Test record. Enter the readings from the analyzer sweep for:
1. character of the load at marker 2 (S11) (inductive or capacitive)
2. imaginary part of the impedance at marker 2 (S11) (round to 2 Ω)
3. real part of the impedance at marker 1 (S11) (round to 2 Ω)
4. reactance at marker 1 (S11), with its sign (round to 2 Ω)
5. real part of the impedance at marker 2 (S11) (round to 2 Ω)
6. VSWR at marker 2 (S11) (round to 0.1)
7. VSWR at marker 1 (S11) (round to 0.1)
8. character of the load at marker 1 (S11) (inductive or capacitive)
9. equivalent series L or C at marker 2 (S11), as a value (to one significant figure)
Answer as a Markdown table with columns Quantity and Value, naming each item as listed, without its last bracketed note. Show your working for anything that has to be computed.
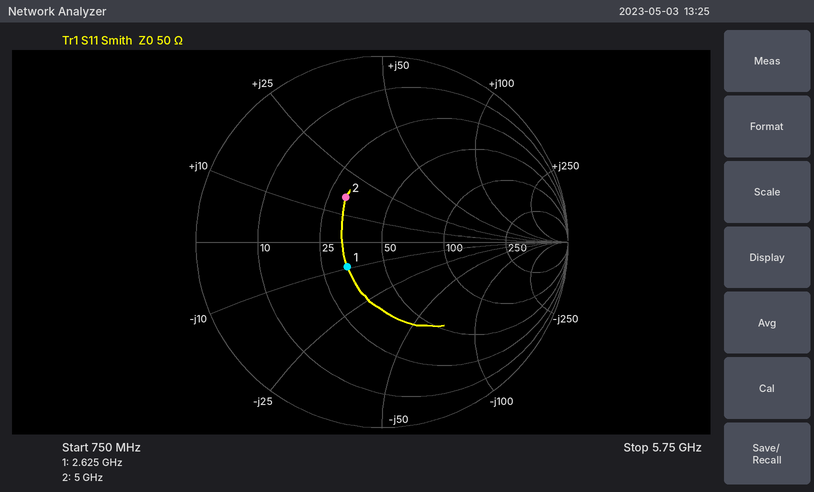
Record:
| Quantity | Value |
|---|---|
| character of the load at marker 2 (S11) | inductive |
| imaginary part of the impedance at marker 2 (S11) | +16 Ω |
| real part of the impedance at marker 1 (S11) | 34 Ω |
| reactance at marker 1 (S11), with its sign | -10 Ω |
| real part of the impedance at marker 2 (S11) | 30 Ω |
| VSWR at marker 2 (S11) | 1.9 |
| VSWR at marker 1 (S11) | 1.6 |
| character of the load at marker 1 (S11) | capacitive |
| equivalent series L or C at marker 2 (S11), as a value | L = 16 Ω/(2π × 5 GHz) ≈ 509 pH, so 500 pH to one significant figure |
